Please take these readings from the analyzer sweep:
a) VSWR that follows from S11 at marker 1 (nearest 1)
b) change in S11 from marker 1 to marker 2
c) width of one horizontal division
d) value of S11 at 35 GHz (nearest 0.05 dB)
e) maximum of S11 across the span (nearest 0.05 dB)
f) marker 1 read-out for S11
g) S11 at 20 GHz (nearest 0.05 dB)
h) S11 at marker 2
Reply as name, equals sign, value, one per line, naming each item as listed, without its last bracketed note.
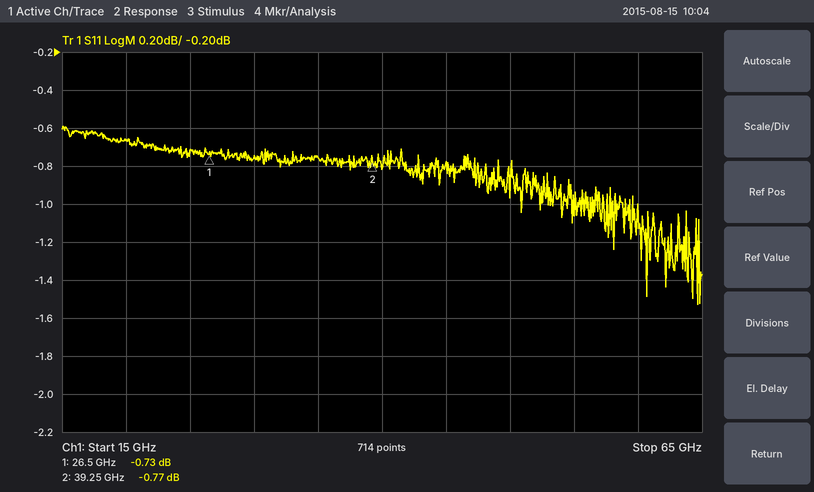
VSWR that follows from S11 at marker 1 = 24
change in S11 from marker 1 to marker 2 = -0.04 dB
width of one horizontal division = 5 GHz
value of S11 at 35 GHz = -0.75 dB
maximum of S11 across the span = -0.60 dB
marker 1 read-out for S11 = -0.73 dB
S11 at 20 GHz = -0.65 dB
S11 at marker 2 = -0.77 dB
